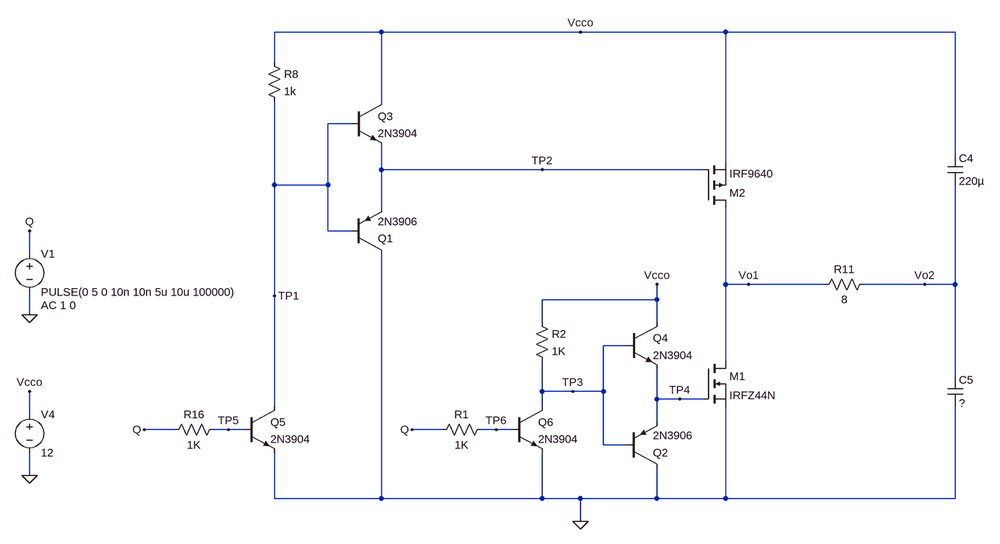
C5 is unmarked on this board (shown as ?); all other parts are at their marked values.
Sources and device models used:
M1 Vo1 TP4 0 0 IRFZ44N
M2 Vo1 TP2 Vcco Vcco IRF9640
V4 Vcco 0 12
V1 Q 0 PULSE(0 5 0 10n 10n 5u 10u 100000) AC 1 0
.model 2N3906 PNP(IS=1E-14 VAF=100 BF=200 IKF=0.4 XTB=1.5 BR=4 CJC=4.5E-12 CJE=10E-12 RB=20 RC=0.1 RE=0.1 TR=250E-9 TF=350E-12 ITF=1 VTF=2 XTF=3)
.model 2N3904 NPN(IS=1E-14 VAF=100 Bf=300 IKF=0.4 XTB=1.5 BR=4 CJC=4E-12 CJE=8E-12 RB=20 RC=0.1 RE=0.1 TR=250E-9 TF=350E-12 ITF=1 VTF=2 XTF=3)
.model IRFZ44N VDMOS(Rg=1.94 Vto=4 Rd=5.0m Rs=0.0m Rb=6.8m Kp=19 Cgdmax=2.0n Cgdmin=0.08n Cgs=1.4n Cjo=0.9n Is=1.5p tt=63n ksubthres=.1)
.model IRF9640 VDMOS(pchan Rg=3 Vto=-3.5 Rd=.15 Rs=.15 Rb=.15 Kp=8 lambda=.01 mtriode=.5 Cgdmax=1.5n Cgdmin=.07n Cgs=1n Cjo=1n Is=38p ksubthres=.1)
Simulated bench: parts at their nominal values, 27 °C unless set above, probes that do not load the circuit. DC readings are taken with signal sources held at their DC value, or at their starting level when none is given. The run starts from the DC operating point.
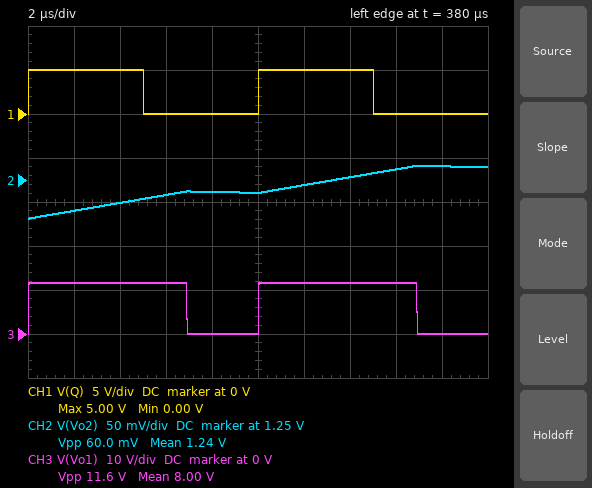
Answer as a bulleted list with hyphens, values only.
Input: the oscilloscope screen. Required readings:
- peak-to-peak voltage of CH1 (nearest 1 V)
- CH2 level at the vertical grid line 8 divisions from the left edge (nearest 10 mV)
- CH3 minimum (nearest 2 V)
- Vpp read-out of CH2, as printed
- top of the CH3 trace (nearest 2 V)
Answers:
- 5 V
- 1.26 V
- 0 V
- 60.0 mV
- 12 V
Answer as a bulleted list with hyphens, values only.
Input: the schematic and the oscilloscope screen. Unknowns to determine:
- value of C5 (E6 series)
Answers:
- 68 µF
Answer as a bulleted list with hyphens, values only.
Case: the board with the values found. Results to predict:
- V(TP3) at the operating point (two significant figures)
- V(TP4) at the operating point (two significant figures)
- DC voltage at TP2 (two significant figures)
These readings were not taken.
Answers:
- 12 V
- 12 V
- 12 V
